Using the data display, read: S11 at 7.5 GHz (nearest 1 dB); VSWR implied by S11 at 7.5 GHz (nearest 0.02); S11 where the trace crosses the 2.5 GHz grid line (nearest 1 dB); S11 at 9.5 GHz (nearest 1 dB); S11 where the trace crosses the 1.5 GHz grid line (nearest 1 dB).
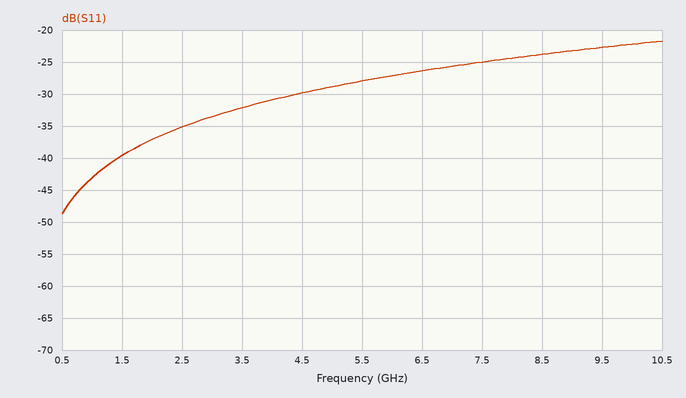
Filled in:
-25 dB
1.12
-35 dB
-23 dB
-40 dB
